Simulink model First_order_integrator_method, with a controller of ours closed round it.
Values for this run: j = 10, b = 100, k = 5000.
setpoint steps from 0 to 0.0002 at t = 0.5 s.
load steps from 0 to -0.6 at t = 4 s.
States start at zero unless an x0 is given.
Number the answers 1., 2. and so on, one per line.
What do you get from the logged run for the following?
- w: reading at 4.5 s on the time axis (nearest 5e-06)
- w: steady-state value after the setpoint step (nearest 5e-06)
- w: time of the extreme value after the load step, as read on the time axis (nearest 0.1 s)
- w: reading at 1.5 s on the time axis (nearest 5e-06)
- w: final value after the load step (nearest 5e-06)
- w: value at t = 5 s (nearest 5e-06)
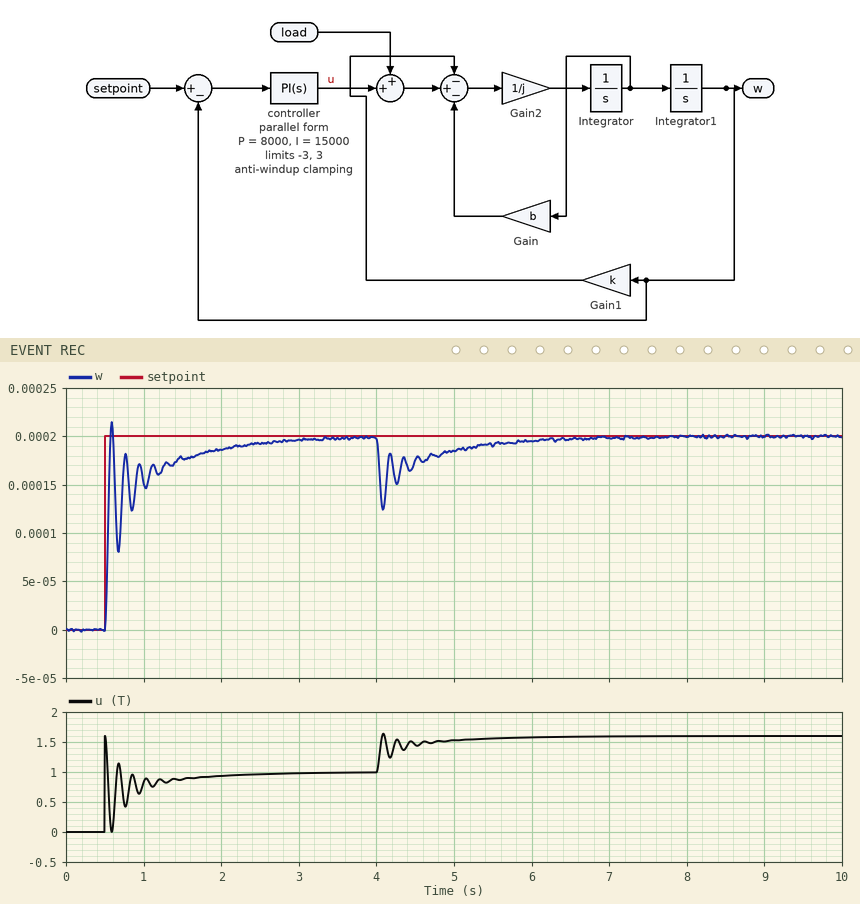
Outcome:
1. 0.000175
2. 0.000200
3. 4.1 s
4. 0.000175
5. 0.000200
6. 0.000185
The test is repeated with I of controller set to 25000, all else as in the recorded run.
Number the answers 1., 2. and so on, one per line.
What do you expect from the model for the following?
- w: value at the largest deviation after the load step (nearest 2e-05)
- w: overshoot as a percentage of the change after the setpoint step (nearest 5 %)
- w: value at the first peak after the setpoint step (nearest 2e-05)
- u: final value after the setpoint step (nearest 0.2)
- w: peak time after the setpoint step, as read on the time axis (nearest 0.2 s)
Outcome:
1. 0.00012
2. 10 %
3. 0.00022
4. 1.0
5. 0.6 s
